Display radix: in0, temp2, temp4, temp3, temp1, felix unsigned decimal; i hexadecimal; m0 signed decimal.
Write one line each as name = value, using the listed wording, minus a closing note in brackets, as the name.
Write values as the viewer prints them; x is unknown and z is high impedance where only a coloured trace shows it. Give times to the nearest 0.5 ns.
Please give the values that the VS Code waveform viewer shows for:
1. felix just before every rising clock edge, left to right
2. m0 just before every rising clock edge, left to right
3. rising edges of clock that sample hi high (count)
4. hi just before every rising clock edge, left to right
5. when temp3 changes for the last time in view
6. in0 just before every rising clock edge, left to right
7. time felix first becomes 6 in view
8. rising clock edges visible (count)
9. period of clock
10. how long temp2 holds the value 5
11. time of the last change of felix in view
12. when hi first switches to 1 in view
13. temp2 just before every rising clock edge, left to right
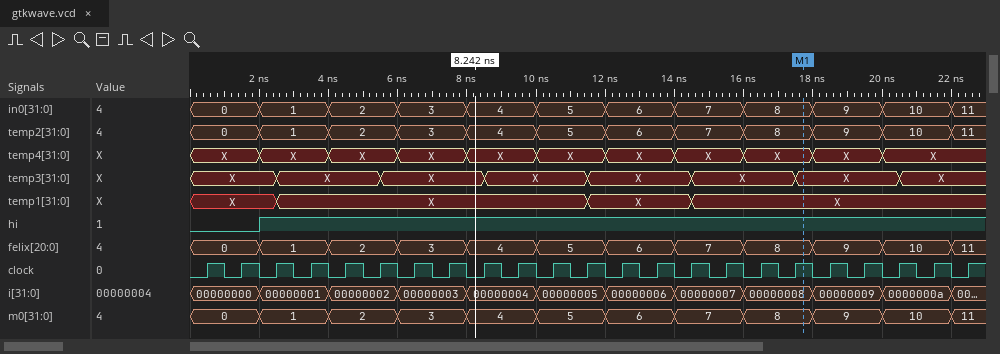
felix just before every rising clock edge, left to right = 0, 0, 1, 1, 2, 2, 3, 3, 4, 4, 5, 5, 6, 6, 7, 7, 8, 8, 9, 9, 10, 10, 11
m0 just before every rising clock edge, left to right = 0, 0, 1, 1, 2, 2, 3, 3, 4, 4, 5, 5, 6, 6, 7, 7, 8, 8, 9, 9, 10, 10, 11
rising edges of clock that sample hi high = 21
hi just before every rising clock edge, left to right = 0 0 1 1 1 1 1 1 1 1 1 1 1 1 1 1 1 1 1 1 1 1 1
when temp3 changes for the last time in view = 20.5 ns
in0 just before every rising clock edge, left to right = 0, 0, 1, 1, 2, 2, 3, 3, 4, 4, 5, 5, 6, 6, 7, 7, 8, 8, 9, 9, 10, 10, 11
time felix first becomes 6 in view = 12 ns
rising clock edges visible = 23
period of clock = 1 ns
how long temp2 holds the value 5 = 2 ns
time of the last change of felix in view = 22 ns
when hi first switches to 1 in view = 2 ns
temp2 just before every rising clock edge, left to right = 0, 0, 1, 1, 2, 2, 3, 3, 4, 4, 5, 5, 6, 6, 7, 7, 8, 8, 9, 9, 10, 10, 11
